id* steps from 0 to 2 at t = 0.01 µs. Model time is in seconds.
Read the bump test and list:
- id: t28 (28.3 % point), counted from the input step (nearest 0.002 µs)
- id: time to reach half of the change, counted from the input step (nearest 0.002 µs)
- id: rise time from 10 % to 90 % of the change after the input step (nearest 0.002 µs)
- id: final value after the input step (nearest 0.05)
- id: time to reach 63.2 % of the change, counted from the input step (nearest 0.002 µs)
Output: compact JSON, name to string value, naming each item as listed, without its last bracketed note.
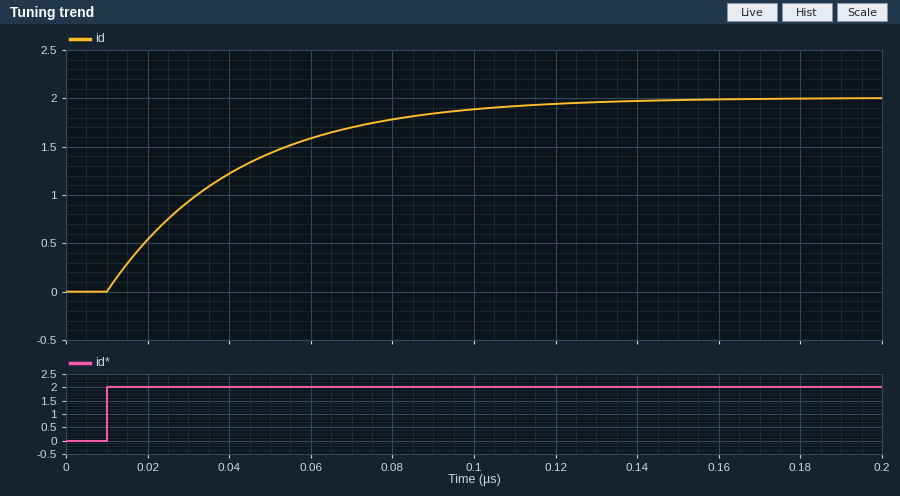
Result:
{"id: t28 (28.3 % point), counted from the input step": "0.010 µs", "id: time to reach half of the change, counted from the input step": "0.022 µs", "id: rise time from 10 % to 90 % of the change after the input step": "0.070 µs", "id: final value after the input step": "2.00", "id: time to reach 63.2 % of the change, counted from the input step": "0.032 µs"}
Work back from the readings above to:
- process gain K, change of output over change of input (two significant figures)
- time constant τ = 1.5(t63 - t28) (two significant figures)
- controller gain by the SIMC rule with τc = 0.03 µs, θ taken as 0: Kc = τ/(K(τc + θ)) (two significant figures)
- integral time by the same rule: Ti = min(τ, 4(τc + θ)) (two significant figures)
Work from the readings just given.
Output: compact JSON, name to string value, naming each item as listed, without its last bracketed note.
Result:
{"process gain K, change of output over change of input": "1.0", "time constant τ = 1.5(t63 - t28)": "0.033 µs", "controller gain by the SIMC rule with τc = 0.03 µs, θ taken as 0: Kc = τ/(K(τc + θ))": "1.1", "integral time by the same rule: Ti = min(τ, 4(τc + θ))": "0.033 µs"}
